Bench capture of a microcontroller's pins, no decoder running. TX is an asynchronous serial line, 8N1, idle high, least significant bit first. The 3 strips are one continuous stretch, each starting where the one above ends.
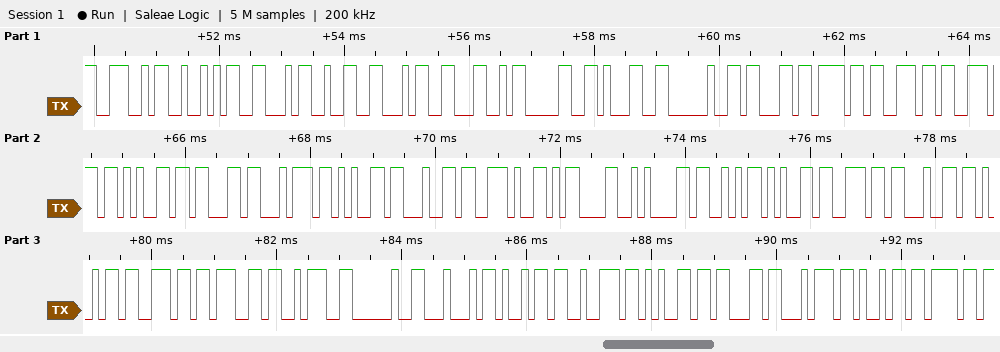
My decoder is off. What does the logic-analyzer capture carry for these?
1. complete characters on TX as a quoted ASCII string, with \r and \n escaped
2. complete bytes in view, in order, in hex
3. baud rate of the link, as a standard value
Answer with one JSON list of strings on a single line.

["\"NRF24L01 connected.\\r\\nSending: Directio\"", "4E 52 46 32 34 4C 30 31 20 63 6F 6E 6E 65 63 74 65 64 2E 0D 0A 53 65 6E 64 69 6E 67 3A 20 44 69 72 65 63 74 69 6F", "9600 baud"]
